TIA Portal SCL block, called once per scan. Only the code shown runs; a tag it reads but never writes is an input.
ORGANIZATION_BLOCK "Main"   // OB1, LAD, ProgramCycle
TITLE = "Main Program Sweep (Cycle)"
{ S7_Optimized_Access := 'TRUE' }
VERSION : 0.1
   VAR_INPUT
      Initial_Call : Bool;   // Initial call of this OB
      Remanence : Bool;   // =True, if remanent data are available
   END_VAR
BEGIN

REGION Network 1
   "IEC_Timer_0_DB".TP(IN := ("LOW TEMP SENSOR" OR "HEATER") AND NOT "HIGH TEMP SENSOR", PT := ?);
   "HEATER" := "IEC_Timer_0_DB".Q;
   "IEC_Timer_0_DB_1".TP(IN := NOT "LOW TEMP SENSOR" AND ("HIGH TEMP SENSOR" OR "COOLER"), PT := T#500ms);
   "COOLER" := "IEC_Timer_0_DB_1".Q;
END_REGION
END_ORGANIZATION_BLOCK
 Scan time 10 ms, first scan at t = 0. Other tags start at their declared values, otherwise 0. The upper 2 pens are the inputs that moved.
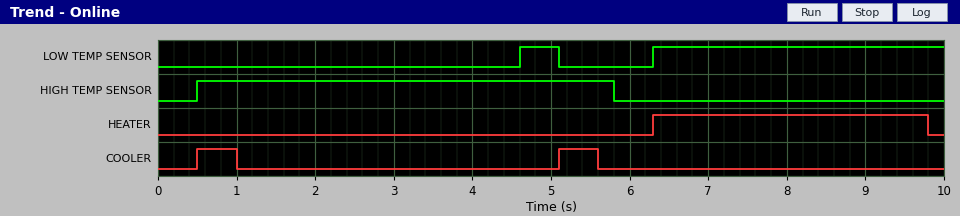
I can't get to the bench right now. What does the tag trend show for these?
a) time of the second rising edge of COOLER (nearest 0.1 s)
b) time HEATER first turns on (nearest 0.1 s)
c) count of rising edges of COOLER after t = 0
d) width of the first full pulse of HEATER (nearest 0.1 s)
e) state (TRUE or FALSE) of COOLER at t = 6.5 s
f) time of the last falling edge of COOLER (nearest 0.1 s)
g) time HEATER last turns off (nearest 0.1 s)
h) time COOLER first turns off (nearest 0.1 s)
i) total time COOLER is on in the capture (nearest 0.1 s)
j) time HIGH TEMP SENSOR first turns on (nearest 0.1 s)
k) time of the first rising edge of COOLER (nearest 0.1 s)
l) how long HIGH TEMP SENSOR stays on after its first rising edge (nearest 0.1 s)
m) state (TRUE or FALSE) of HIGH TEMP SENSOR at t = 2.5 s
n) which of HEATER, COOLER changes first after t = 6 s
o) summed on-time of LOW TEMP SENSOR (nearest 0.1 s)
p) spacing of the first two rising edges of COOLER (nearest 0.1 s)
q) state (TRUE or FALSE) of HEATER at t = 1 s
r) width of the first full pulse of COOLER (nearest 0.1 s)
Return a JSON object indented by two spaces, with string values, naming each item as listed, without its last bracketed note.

{
  "time of the second rising edge of COOLER": "5.1 s",
  "time HEATER first turns on": "6.3 s",
  "count of rising edges of COOLER after t = 0": "2",
  "width of the first full pulse of HEATER": "3.5 s",
  "state (TRUE or FALSE) of COOLER at t = 6.5 s": "FALSE",
  "time of the last falling edge of COOLER": "5.6 s",
  "time HEATER last turns off": "9.8 s",
  "time COOLER first turns off": "1.0 s",
  "total time COOLER is on in the capture": "1.0 s",
  "time HIGH TEMP SENSOR first turns on": "0.5 s",
  "time of the first rising edge of COOLER": "0.5 s",
  "how long HIGH TEMP SENSOR stays on after its first rising edge": "5.3 s",
  "state (TRUE or FALSE) of HIGH TEMP SENSOR at t = 2.5 s": "TRUE",
  "which of HEATER, COOLER changes first after t = 6 s": "HEATER",
  "summed on-time of LOW TEMP SENSOR": "4.2 s",
  "spacing of the first two rising edges of COOLER": "4.6 s",
  "state (TRUE or FALSE) of HEATER at t = 1 s": "FALSE",
  "width of the first full pulse of COOLER": "0.5 s"
}
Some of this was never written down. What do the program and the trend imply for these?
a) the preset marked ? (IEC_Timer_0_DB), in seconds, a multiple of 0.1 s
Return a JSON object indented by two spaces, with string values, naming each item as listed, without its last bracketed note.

{
  "the preset marked ? (IEC_Timer_0_DB), in seconds, a multiple of 0.1 s": "3.5 s"
}
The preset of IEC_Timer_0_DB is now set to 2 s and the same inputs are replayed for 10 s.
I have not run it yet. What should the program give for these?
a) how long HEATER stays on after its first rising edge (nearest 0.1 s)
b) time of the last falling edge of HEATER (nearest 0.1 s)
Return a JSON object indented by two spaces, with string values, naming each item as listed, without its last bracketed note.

{
  "how long HEATER stays on after its first rising edge": "2.0 s",
  "time of the last falling edge of HEATER": "8.3 s"
}
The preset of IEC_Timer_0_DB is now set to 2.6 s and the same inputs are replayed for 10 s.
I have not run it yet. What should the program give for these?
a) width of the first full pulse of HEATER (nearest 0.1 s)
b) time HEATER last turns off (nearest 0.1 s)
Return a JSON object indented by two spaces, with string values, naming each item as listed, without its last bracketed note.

{
  "width of the first full pulse of HEATER": "2.6 s",
  "time HEATER last turns off": "8.9 s"
}
